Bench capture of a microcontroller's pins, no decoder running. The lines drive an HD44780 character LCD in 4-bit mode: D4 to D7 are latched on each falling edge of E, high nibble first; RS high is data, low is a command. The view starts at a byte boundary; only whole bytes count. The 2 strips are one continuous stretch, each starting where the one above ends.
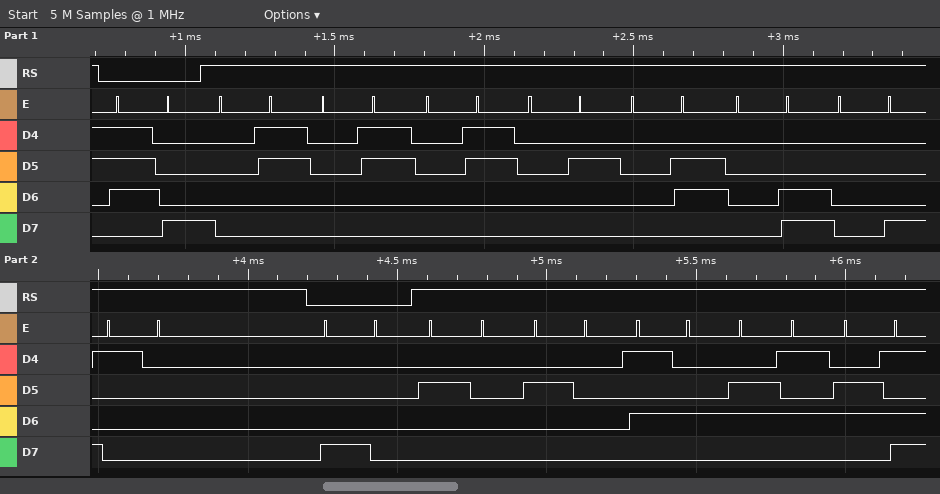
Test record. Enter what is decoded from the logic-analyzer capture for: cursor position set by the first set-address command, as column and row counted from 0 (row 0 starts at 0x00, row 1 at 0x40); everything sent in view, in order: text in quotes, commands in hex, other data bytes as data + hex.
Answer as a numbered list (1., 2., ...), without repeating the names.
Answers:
1. column 0, row 0
2. 0x78 data 03 03 03 02 06 0C 08 10 0x80 "  Tem"
